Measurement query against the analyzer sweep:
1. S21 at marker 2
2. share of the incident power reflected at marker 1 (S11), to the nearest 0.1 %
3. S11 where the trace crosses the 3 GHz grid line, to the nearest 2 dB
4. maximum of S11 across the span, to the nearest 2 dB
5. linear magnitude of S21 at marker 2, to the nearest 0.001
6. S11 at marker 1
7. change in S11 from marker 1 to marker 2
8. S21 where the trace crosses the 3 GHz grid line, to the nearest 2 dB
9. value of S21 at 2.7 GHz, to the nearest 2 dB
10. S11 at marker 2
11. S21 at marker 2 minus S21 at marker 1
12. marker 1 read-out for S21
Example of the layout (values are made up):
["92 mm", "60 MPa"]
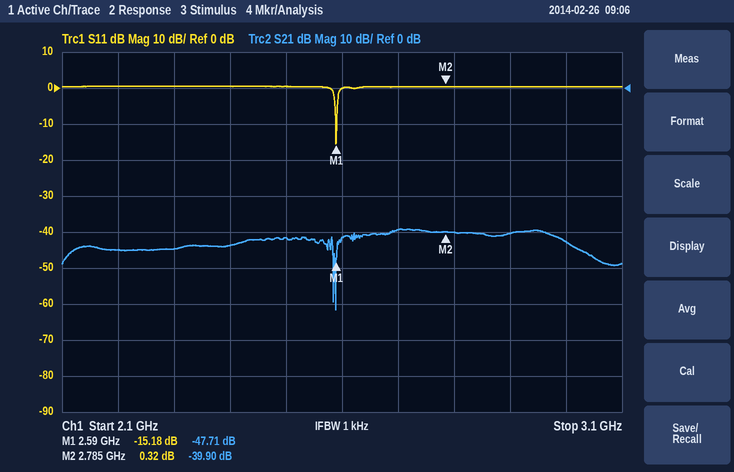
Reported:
["-39.90 dB", "3.0 %", "0 dB", "0 dB", "0.010", "-15.18 dB", "15.50 dB", "-42 dB", "-40 dB", "0.32 dB", "7.81 dB", "-47.71 dB"]
